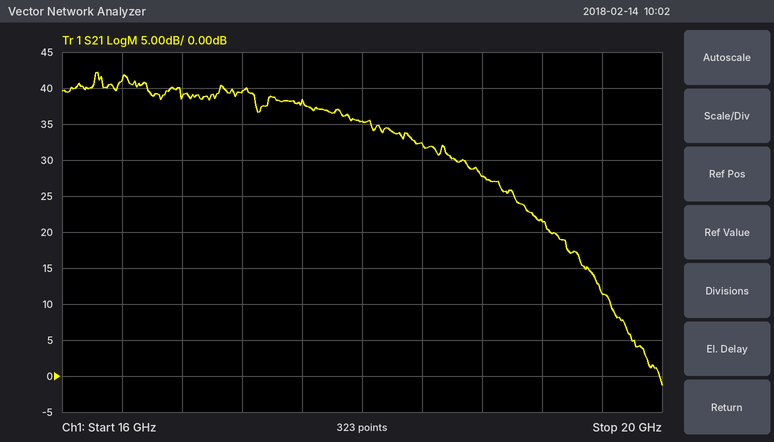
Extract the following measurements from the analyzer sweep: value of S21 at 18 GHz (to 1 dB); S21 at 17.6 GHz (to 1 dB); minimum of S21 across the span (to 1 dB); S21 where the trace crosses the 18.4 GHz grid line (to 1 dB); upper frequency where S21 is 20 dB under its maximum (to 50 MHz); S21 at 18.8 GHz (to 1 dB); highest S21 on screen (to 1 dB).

35 dB
38 dB
-1 dB
32 dB
19.15 GHz
28 dB
42 dB
